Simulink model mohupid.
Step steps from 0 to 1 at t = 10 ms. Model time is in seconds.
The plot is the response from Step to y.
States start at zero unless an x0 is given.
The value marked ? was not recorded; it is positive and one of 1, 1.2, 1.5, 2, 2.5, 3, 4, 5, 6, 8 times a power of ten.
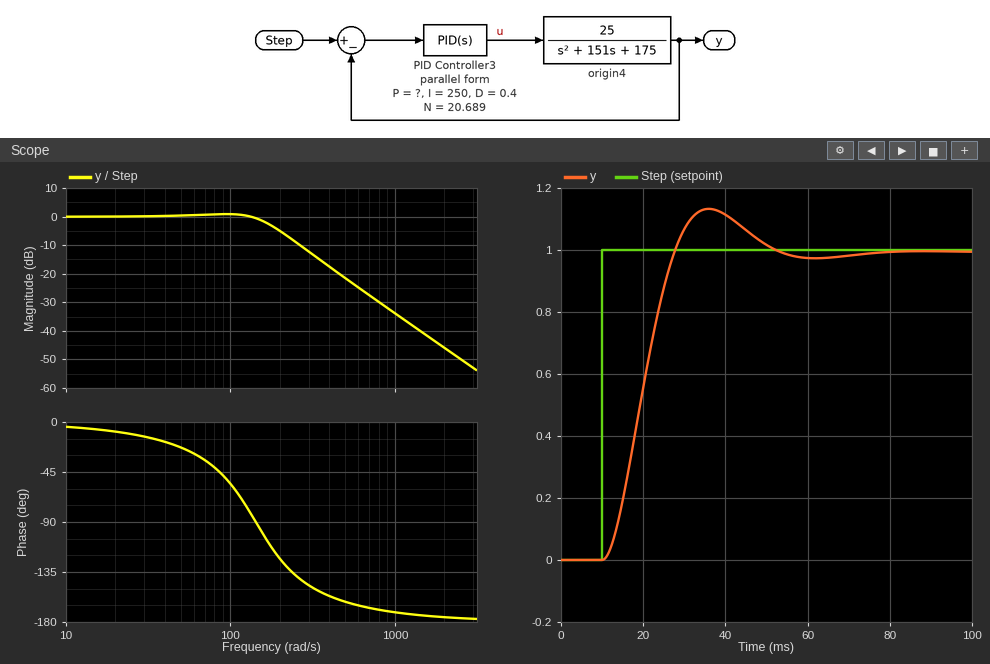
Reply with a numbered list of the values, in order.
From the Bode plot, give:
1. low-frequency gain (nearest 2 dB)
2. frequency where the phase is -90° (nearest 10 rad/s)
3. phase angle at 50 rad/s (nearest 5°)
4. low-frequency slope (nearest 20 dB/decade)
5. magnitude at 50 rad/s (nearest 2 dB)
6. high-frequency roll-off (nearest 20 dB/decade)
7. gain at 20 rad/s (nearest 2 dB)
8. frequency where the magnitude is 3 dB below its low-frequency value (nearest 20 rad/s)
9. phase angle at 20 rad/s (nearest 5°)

1. 0 dB
2. 140 rad/s
3. -25°
4. 0 dB/decade
5. 0 dB
6. -40 dB/decade
7. 0 dB
8. 180 rad/s
9. -10°
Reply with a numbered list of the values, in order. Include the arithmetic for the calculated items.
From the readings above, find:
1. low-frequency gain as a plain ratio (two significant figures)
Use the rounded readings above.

1. 10^(0 / 20) = 1.0
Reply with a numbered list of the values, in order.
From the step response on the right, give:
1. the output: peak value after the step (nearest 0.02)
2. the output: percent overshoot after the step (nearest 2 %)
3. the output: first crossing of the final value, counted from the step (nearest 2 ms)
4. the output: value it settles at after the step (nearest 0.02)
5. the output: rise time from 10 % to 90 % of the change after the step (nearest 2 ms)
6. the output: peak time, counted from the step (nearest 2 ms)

1. 1.14
2. 14 %
3. 18 ms
4. 1.00
5. 12 ms
6. 26 ms
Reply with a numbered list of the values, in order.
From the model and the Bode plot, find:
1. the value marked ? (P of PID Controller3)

1. 800
